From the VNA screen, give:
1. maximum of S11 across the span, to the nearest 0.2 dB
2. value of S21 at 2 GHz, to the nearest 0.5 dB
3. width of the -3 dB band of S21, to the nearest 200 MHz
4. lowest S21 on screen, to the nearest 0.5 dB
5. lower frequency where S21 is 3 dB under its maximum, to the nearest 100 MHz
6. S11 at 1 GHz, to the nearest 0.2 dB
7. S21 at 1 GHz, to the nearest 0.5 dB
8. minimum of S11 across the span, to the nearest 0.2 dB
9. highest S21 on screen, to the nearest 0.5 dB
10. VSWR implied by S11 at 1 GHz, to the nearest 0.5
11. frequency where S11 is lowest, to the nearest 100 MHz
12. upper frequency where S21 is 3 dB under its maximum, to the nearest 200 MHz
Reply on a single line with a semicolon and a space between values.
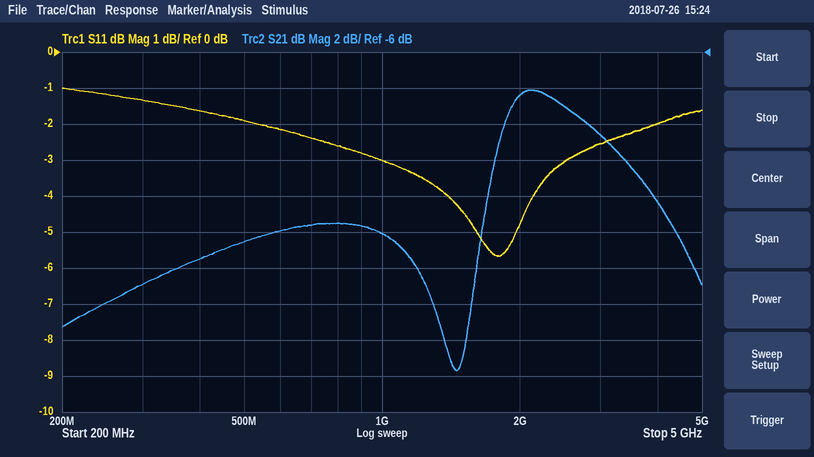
-1.0 dB; -8.5 dB; 1.4 GHz; -23.5 dB; 1.8 GHz; -3.0 dB; -16.0 dB; -5.6 dB; -8.0 dB; 6.0; 1.8 GHz; 3.2 GHz
